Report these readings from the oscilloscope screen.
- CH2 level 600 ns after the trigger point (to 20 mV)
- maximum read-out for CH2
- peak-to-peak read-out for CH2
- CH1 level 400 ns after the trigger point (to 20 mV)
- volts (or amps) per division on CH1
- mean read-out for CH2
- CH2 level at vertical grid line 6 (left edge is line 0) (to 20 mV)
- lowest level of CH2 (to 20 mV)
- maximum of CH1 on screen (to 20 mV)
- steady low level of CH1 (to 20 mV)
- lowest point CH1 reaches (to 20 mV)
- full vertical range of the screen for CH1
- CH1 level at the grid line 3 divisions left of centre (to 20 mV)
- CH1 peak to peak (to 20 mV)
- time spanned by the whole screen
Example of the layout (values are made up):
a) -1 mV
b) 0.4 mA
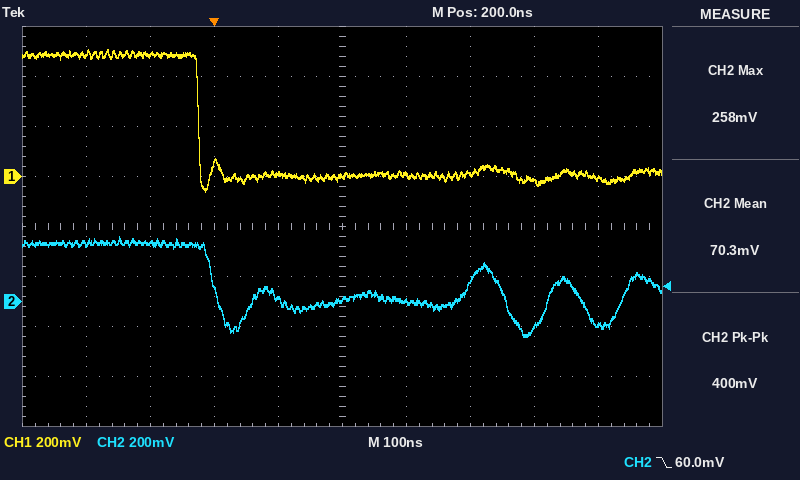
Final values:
a) -100 mV
b) 258 mV
c) 400 mV
d) 20 mV
e) 200 mV
f) 70.3 mV
g) 0 mV
h) -140 mV
i) 500 mV
j) 0 mV
k) -60 mV
l) 1.6 V
m) 480 mV
n) 560 mV
o) 1 µs
